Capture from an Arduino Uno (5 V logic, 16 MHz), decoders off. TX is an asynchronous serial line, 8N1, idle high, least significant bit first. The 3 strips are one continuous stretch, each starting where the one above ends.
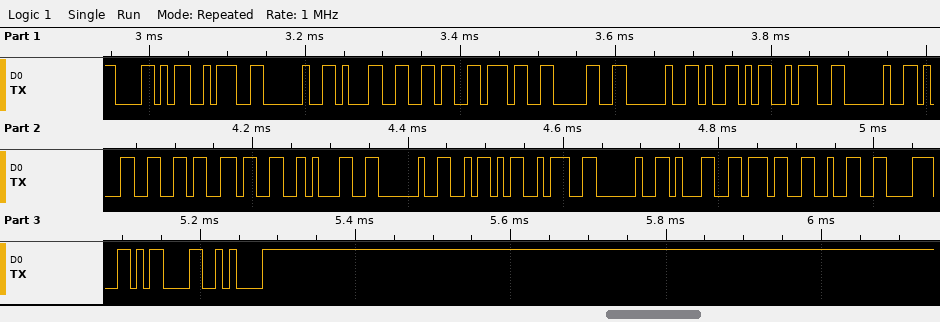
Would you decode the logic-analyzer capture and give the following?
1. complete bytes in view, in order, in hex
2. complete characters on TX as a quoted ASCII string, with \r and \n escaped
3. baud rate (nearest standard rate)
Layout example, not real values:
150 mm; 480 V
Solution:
58 3A 20 31 36 37 30 20 59 3A 20 31 36 33 31 20 5A 3A 20 31 37 32 38 0D 0A; "X: 1670 Y: 1631 Z: 1728\r\n"; 115200 baud
